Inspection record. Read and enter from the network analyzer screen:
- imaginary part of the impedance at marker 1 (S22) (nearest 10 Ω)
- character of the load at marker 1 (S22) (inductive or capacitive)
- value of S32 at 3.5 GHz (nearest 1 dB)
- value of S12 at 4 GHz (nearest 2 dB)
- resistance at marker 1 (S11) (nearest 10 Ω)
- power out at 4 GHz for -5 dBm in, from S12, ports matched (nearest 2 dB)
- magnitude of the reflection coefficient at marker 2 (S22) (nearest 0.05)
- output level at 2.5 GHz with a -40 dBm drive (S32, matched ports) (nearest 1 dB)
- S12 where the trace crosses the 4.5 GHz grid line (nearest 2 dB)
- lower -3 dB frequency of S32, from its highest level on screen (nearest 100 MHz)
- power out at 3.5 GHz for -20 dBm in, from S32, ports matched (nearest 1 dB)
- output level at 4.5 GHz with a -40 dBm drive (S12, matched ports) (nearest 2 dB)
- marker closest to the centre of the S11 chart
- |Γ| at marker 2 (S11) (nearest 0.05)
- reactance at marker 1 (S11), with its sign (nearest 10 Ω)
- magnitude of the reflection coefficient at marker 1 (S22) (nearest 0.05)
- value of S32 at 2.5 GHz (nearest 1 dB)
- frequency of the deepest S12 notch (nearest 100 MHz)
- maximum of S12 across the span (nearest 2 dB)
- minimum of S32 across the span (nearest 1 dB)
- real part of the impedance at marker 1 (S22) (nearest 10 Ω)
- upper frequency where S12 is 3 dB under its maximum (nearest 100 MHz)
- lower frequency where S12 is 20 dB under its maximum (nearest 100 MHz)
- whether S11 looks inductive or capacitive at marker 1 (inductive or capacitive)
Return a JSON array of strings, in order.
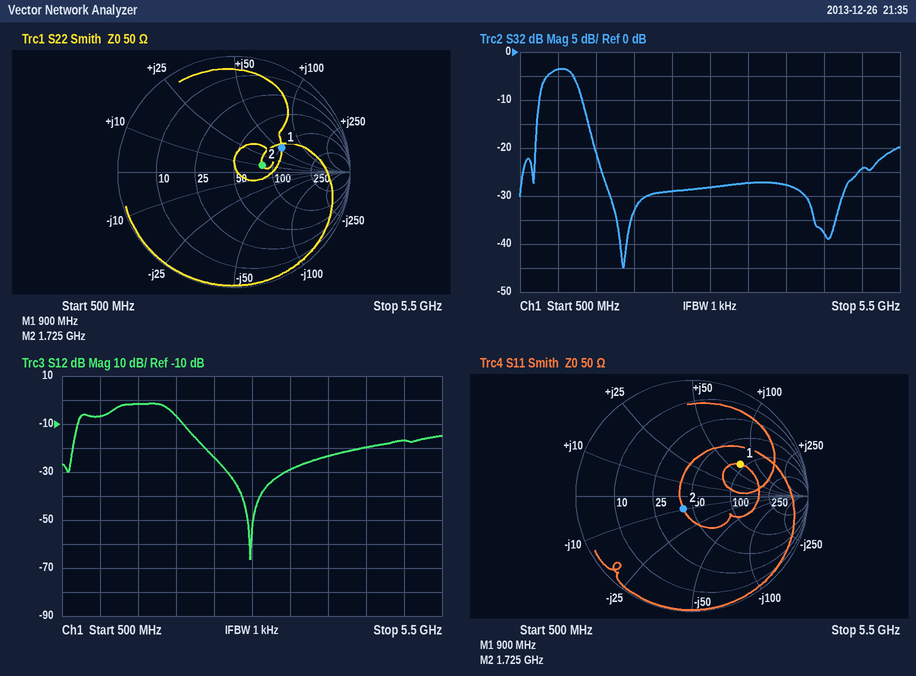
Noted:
["+50 Ω", "inductive", "-27 dB", "-24 dB", "90 Ω", "-28 dBm", "0.25", "-69 dBm", "-20 dB", "800 MHz", "-47 dBm", "-60 dBm", "marker 2", "0.15", "+70 Ω", "0.45", "-29 dB", "3.0 GHz", "-2 dB", "-45 dB", "100 Ω", "1.9 GHz", "600 MHz", "inductive"]
